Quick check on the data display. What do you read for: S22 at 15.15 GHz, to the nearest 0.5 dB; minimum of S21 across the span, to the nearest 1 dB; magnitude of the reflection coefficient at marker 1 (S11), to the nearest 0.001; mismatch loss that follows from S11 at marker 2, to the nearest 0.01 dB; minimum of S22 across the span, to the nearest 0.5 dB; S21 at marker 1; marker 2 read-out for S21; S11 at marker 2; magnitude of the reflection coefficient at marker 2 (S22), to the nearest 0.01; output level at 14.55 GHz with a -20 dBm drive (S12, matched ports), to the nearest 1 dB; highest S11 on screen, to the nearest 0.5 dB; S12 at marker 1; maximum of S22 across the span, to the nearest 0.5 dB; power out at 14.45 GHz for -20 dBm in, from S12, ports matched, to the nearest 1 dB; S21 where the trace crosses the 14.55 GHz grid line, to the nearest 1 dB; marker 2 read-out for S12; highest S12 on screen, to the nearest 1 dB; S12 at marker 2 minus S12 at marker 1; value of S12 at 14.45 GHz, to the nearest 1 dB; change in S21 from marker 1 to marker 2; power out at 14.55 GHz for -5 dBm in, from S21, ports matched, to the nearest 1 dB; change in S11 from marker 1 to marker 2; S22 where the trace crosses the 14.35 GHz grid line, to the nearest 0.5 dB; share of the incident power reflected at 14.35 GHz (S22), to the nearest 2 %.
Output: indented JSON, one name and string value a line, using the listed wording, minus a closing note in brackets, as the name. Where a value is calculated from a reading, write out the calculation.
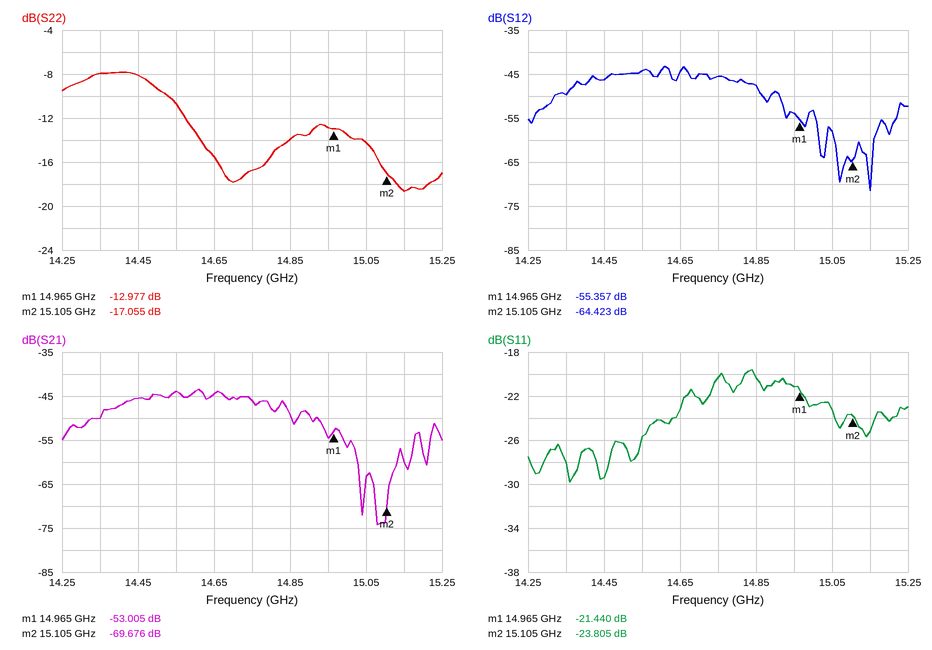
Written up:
{
  "S22 at 15.15 GHz, to the nearest 0.5 dB": "-18.5 dB",
  "minimum of S21 across the span, to the nearest 1 dB": "-74 dB",
  "magnitude of the reflection coefficient at marker 1 (S11), to the nearest 0.001": "10^(-21.44/20) ≈ 0.085",
  "mismatch loss that follows from S11 at marker 2, to the nearest 0.01 dB": "−10 log10(1 − 10^(-23.805/10)) ≈ 0.02 dB",
  "minimum of S22 across the span, to the nearest 0.5 dB": "-18.5 dB",
  "S21 at marker 1": "-53.005 dB",
  "marker 2 read-out for S21": "-69.676 dB",
  "S11 at marker 2": "-23.805 dB",
  "magnitude of the reflection coefficient at marker 2 (S22), to the nearest 0.01": "10^(-17.055/20) ≈ 0.14",
  "output level at 14.55 GHz with a -20 dBm drive (S12, matched ports), to the nearest 1 dB": "-20 dBm + (-44 dB) = -64 dBm",
  "highest S11 on screen, to the nearest 0.5 dB": "-19.5 dB",
  "S12 at marker 1": "-55.357 dB",
  "maximum of S22 across the span, to the nearest 0.5 dB": "-8.0 dB",
  "power out at 14.45 GHz for -20 dBm in, from S12, ports matched, to the nearest 1 dB": "-20 dBm + (-46 dB) = -66 dBm",
  "S21 where the trace crosses the 14.55 GHz grid line, to the nearest 1 dB": "-44 dB",
  "marker 2 read-out for S12": "-64.423 dB",
  "highest S12 on screen, to the nearest 1 dB": "-43 dB",
  "S12 at marker 2 minus S12 at marker 1": "-64.423 − (-55.357) = -9.066 dB",
  "value of S12 at 14.45 GHz, to the nearest 1 dB": "-46 dB",
  "change in S21 from marker 1 to marker 2": "-69.676 − (-53.005) = -16.671 dB",
  "power out at 14.55 GHz for -5 dBm in, from S21, ports matched, to the nearest 1 dB": "-5 dBm + (-44 dB) = -49 dBm",
  "change in S11 from marker 1 to marker 2": "-23.805 − (-21.44) = -2.365 dB",
  "S22 where the trace crosses the 14.35 GHz grid line, to the nearest 0.5 dB": "-8.0 dB",
  "share of the incident power reflected at 14.35 GHz (S22), to the nearest 2 %": "10^(-8/10) ≈ 16 %"
}
